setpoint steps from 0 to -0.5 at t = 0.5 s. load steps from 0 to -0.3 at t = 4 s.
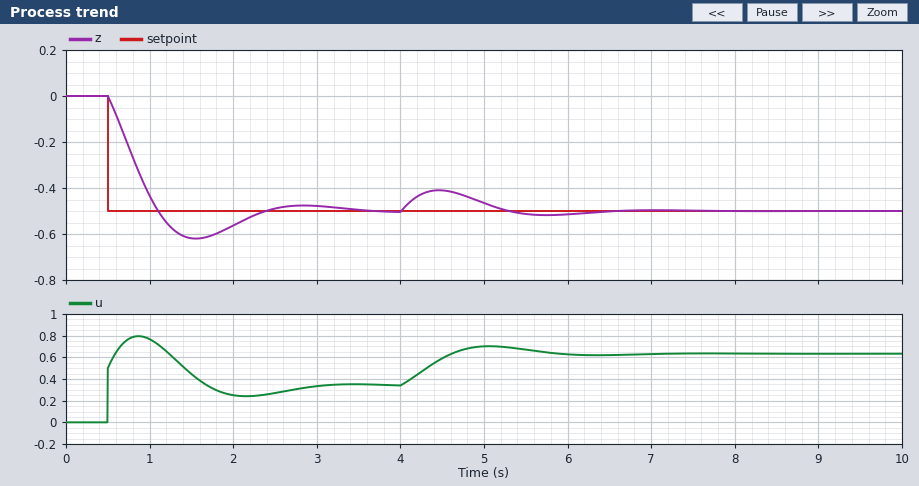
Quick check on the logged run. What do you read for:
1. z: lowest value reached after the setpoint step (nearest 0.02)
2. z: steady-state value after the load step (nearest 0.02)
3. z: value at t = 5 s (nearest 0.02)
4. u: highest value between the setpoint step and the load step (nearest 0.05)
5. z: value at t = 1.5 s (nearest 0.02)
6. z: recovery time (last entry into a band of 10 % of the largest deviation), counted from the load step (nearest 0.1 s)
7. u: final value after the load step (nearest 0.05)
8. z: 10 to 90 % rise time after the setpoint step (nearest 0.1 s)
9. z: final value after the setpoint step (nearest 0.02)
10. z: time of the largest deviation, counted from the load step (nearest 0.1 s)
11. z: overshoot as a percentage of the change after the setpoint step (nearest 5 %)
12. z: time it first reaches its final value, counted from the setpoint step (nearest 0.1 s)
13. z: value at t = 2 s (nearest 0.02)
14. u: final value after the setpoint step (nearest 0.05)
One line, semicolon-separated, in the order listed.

-0.62; -0.50; -0.46; 0.80; -0.62; 2.2 s; 0.65; 0.5 s; -0.50; 0.5 s; 25 %; 0.6 s; -0.56; 0.35
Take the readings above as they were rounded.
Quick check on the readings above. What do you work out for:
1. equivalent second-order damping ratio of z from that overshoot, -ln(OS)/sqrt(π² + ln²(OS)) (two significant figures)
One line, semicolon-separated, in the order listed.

0.40
